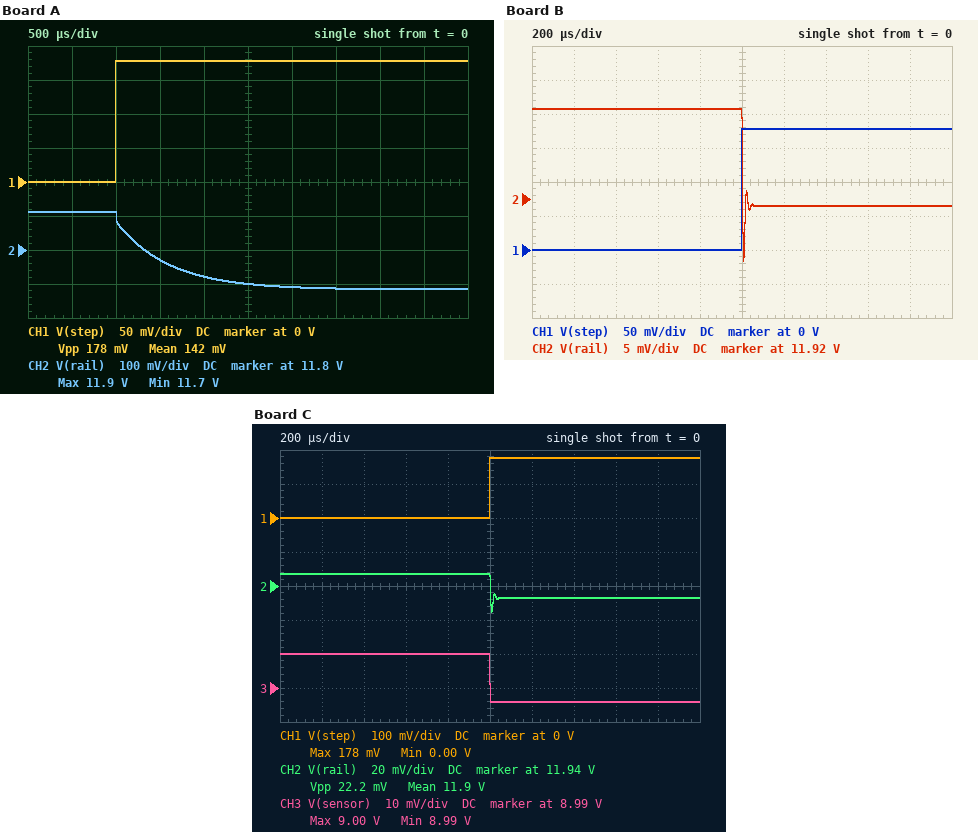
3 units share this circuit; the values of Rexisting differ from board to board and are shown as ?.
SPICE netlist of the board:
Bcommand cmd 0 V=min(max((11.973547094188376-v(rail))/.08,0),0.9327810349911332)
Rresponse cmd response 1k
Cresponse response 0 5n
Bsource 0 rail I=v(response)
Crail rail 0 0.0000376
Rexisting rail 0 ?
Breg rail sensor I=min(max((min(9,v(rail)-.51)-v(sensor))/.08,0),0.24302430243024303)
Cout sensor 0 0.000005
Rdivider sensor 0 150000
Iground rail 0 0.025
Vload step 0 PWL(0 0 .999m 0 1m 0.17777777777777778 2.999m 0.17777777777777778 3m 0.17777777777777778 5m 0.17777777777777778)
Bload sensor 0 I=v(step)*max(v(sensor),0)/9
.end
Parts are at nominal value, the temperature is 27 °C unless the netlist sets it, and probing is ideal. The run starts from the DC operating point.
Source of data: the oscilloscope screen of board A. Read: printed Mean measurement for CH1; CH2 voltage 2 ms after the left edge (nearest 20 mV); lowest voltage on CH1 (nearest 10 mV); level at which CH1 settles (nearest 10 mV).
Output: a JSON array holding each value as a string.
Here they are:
["142 mV", "11.72 V", "0 V", "180 mV"]
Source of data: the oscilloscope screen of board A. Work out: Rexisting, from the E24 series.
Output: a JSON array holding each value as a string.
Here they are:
["16 Ω"]
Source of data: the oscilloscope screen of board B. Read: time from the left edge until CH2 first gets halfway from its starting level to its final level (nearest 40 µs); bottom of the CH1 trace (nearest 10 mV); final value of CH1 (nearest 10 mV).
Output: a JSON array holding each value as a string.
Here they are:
["1.00 ms", "0 V", "180 mV"]
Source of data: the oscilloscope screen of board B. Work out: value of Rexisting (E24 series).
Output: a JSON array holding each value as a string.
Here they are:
["22 Ω"]
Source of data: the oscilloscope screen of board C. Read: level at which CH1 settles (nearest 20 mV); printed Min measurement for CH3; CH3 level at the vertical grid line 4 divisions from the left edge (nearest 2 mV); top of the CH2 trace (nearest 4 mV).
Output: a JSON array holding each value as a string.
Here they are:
["180 mV", "8.99 V", "9.000 V", "11.948 V"]
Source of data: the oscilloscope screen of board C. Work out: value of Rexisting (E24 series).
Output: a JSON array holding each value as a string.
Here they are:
["39 Ω"]
